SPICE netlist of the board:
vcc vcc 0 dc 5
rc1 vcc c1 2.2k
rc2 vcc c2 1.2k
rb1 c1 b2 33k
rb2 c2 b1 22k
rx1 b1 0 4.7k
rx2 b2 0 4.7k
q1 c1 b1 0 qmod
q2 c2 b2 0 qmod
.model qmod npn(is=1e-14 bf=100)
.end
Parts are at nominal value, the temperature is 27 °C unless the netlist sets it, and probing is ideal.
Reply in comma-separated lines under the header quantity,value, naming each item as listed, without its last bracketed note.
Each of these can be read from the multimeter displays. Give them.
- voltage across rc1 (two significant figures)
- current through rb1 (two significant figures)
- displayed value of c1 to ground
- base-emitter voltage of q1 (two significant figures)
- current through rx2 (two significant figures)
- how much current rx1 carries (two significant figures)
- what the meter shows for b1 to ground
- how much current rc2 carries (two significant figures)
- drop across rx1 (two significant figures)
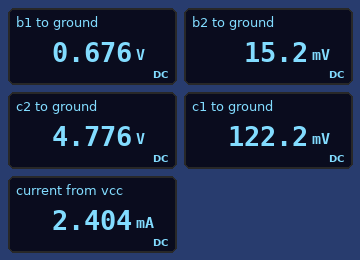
quantity,value
voltage across rc1,4.9 V
current through rb1,3.2 µA
displayed value of c1 to ground,122.2 mV
base-emitter voltage of q1,680 mV
current through rx2,3.2 µA
how much current rx1 carries,140 µA
what the meter shows for b1 to ground,0.676 V
how much current rc2 carries,190 µA
drop across rx1,680 mV
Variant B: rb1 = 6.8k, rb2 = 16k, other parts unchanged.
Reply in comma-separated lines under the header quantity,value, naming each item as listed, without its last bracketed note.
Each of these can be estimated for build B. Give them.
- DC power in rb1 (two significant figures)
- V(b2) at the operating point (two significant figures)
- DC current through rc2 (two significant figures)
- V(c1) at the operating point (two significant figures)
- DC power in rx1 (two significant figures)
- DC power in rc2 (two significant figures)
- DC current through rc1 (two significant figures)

quantity,value
DC power in rb1,160 µW
V(b2) at the operating point,660 mV
DC current through rc2,1.6 mA
V(c1) at the operating point,1.7 V
DC power in rx1,93 µW
DC power in rc2,2.9 mW
DC current through rc1,1.5 mA
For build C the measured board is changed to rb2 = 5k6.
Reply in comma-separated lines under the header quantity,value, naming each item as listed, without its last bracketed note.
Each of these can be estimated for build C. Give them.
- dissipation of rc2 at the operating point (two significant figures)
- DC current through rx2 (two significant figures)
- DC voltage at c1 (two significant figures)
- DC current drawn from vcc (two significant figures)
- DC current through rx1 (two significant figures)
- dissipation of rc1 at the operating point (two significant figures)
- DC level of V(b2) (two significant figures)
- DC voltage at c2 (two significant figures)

quantity,value
dissipation of rc2 at the operating point,480 µW
DC current through rx2,1.3 µA
DC voltage at c1,50 mV
DC current drawn from vcc,2.9 mA
DC current through rx1,150 µA
dissipation of rc1 at the operating point,11 mW
DC level of V(b2),6.2 mV
DC voltage at c2,4.2 V
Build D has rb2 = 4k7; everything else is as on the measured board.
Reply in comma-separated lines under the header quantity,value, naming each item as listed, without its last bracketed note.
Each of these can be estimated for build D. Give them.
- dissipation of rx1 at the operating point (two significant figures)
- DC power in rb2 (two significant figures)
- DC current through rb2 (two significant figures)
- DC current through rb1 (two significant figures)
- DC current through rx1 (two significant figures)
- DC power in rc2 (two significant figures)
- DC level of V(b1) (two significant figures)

quantity,value
dissipation of rx1 at the operating point,100 µW
DC power in rb2,2.5 mW
DC current through rb2,730 µA
DC current through rb1,1.2 µA
DC current through rx1,150 µA
DC power in rc2,640 µW
DC level of V(b1),690 mV
